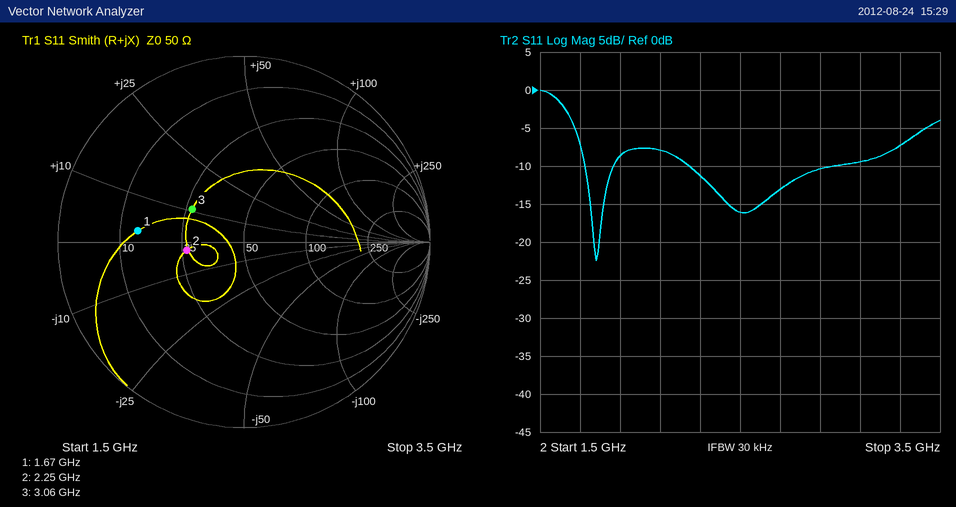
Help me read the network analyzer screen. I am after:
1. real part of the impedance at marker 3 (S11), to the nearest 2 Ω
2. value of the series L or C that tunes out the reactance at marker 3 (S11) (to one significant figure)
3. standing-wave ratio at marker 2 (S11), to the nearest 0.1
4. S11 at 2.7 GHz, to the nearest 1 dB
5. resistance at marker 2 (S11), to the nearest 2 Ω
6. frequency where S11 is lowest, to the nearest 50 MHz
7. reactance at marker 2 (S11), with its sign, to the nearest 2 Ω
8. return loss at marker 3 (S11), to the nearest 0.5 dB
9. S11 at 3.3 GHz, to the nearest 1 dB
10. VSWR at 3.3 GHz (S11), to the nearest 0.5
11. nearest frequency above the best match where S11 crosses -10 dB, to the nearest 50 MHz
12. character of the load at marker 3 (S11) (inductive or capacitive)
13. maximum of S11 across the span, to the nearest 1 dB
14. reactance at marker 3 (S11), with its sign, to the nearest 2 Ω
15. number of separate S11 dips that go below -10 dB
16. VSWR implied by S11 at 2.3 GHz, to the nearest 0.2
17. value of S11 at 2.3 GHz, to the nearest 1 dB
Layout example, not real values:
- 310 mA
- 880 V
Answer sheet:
- 26 Ω
- 5 pF
- 1.9
- -13 dB
- 26 Ω
- 1.80 GHz
- -2 Ω
- 9.5 dB
- -7 dB
- 2.5
- 1.85 GHz
- inductive
- 0 dB
- +10 Ω
- 2
- 1.8
- -11 dB
